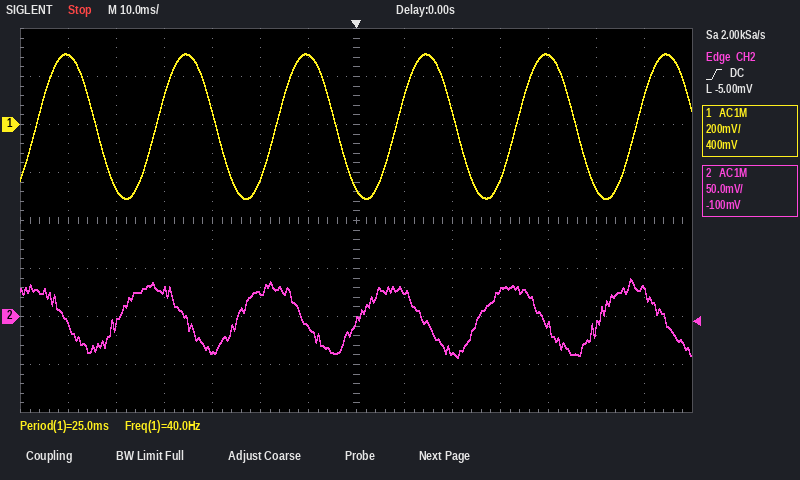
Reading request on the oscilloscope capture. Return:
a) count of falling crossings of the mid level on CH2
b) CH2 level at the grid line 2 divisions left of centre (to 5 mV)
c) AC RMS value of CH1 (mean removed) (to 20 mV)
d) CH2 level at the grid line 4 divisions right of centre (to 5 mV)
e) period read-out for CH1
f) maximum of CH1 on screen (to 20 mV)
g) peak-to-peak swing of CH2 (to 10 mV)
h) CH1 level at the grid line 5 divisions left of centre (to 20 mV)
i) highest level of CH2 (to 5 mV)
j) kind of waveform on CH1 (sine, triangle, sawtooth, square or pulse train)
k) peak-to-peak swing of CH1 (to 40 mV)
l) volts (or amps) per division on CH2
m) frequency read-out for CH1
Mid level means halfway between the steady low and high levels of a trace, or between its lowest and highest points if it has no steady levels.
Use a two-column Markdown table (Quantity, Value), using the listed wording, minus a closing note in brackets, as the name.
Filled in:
| Quantity | Value |
|---|---|
| count of falling crossings of the mid level on CH2 | 6 |
| CH2 level at the grid line 2 divisions left of centre | 25 mV |
| AC RMS value of CH1 (mean removed) | 220 mV |
| CH2 level at the grid line 4 divisions right of centre | -10 mV |
| period read-out for CH1 | 25.0 ms |
| maximum of CH1 on screen | 300 mV |
| peak-to-peak swing of CH2 | 80 mV |
| CH1 level at the grid line 5 divisions left of centre | -260 mV |
| highest level of CH2 | 40 mV |
| kind of waveform on CH1 | sine |
| peak-to-peak swing of CH1 | 600 mV |
| volts (or amps) per division on CH2 | 50 mV |
| frequency read-out for CH1 | 40.0 Hz |
